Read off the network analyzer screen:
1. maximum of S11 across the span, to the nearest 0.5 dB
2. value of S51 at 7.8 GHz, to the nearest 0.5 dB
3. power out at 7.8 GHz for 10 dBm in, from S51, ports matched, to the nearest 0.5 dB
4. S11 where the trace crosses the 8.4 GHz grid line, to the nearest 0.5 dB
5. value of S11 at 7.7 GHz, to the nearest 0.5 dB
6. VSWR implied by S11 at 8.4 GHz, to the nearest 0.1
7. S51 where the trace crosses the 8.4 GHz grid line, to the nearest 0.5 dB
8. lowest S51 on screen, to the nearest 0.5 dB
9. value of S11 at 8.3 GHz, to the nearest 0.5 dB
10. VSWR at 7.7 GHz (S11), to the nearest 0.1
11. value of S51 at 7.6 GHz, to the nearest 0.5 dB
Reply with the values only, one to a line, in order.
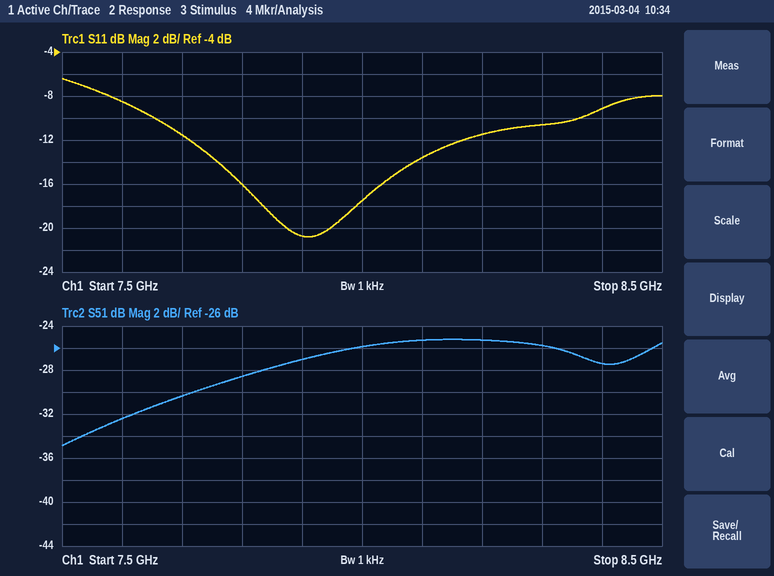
-6.5 dB
-28.5 dB
-18.5 dBm
-9.0 dB
-11.5 dB
2.1
-27.5 dB
-35.0 dB
-10.5 dB
1.7
-32.5 dB
